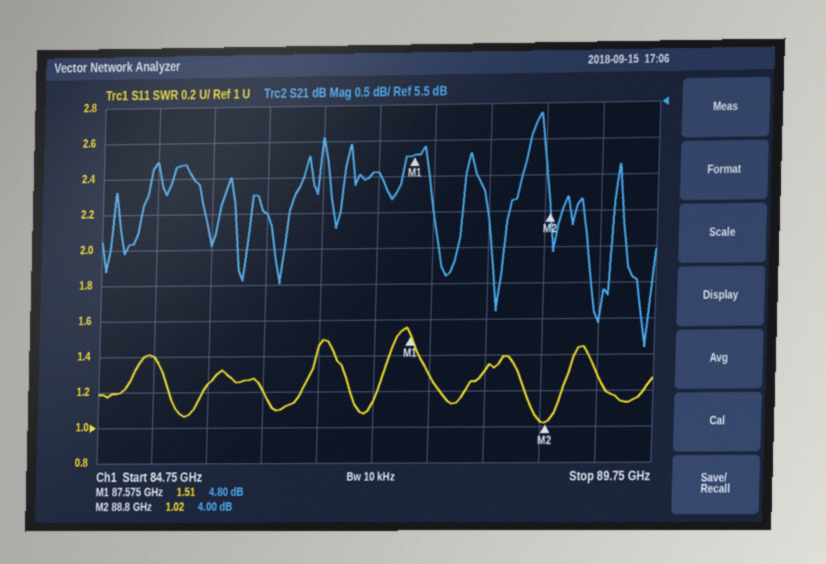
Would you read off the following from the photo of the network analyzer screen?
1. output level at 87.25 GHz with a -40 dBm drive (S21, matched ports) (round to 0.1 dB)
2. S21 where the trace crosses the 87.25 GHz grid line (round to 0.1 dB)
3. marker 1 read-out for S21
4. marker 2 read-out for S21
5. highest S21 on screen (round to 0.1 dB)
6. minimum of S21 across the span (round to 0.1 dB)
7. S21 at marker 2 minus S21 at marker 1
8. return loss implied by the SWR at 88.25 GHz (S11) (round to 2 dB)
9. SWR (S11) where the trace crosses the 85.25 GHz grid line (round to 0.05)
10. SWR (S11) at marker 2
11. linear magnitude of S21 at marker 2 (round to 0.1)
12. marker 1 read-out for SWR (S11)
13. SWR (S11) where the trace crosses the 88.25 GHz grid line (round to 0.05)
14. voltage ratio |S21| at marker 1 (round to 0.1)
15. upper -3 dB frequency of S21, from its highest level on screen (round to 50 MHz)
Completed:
-35.4 dBm
4.6 dB
4.80 dB
4.00 dB
5.4 dB
2.1 dB
-0.80 dB
18 dB
1.40
1.02
1.6
1.51
1.30
1.7
89.65 GHz
